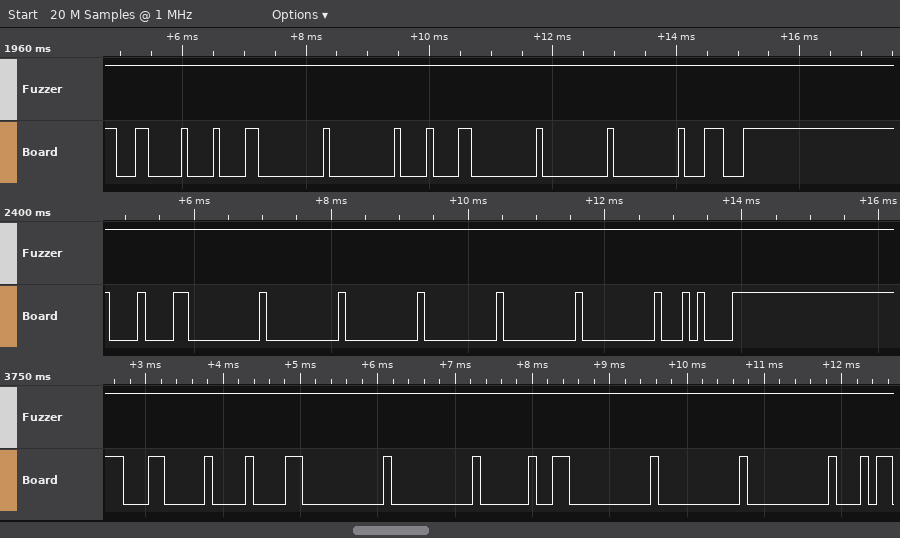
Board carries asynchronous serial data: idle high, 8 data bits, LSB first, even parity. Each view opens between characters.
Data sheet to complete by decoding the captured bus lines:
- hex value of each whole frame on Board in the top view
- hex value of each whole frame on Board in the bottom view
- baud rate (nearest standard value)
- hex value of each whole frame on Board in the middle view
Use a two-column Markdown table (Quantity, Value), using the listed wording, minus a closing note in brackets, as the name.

| Quantity | Value |
|---|---|
| hex value of each whole frame on Board in the top view | 0C, 08, 00, 00, 08, 00, 00, 00, 1C |
| hex value of each whole frame on Board in the bottom view | 0C, 08, 00, 00, 20, 00, 00, 00 |
| baud rate | 9600 baud |
| hex value of each whole frame on Board in the middle view | 08, 00, 00, 00, 00, 00, 00, 14 |
